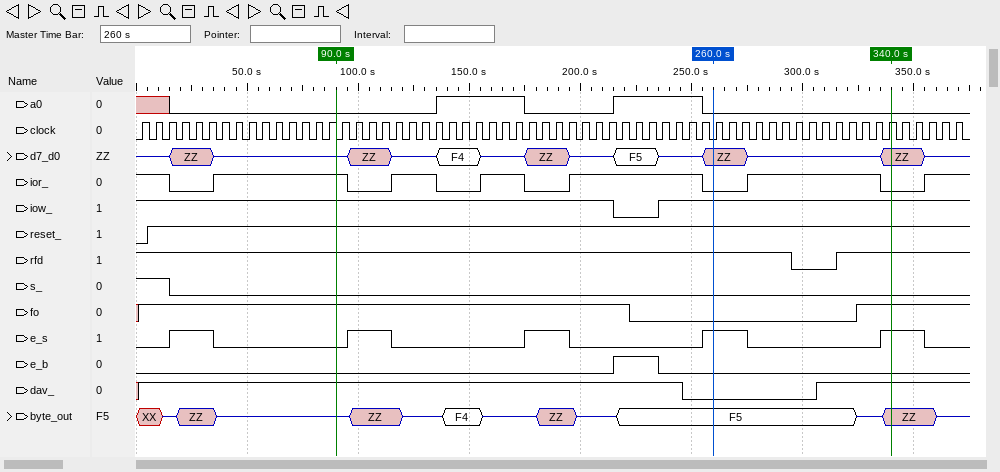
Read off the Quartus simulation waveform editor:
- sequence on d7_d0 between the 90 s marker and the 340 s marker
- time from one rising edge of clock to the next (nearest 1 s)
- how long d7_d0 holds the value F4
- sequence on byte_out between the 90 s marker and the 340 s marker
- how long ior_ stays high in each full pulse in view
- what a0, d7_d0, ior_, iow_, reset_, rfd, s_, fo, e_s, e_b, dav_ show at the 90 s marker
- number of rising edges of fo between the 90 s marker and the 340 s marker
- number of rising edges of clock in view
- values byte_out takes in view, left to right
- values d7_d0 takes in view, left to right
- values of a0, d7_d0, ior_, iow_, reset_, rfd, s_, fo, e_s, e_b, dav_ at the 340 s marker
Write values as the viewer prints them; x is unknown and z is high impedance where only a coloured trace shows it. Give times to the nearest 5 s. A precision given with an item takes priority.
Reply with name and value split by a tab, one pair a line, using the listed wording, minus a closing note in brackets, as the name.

sequence on d7_d0 between the 90 s marker and the 340 s marker	z, ZZ, z, F4, z, ZZ, z, F5, z, ZZ, z, ZZ
time from one rising edge of clock to the next	6 s
how long d7_d0 holds the value F4	20 s
sequence on byte_out between the 90 s marker and the 340 s marker	z, ZZ, z, F4, z, ZZ, z, F5, z, ZZ
how long ior_ stays high in each full pulse in view	60 s, 20 s, 20 s, 60 s, 60 s
what a0, d7_d0, ior_, iow_, reset_, rfd, s_, fo, e_s, e_b, dav_ show at the 90 s marker	a0=0, d7_d0=z, ior_=1, iow_=1, reset_=1, rfd=1, s_=0, fo=1, e_s=0, e_b=0, dav_=1
number of rising edges of fo between the 90 s marker and the 340 s marker	1
number of rising edges of clock in view	62
values byte_out takes in view, left to right	XX, z, ZZ, z, ZZ, z, F4, z, ZZ, z, F5, z, ZZ, z
values d7_d0 takes in view, left to right	z, ZZ, z, ZZ, z, F4, z, ZZ, z, F5, z, ZZ, z, ZZ, z
values of a0, d7_d0, ior_, iow_, reset_, rfd, s_, fo, e_s, e_b, dav_ at the 340 s marker	a0=0, d7_d0=ZZ, ior_=0, iow_=1, reset_=1, rfd=1, s_=0, fo=1, e_s=1, e_b=0, dav_=1
